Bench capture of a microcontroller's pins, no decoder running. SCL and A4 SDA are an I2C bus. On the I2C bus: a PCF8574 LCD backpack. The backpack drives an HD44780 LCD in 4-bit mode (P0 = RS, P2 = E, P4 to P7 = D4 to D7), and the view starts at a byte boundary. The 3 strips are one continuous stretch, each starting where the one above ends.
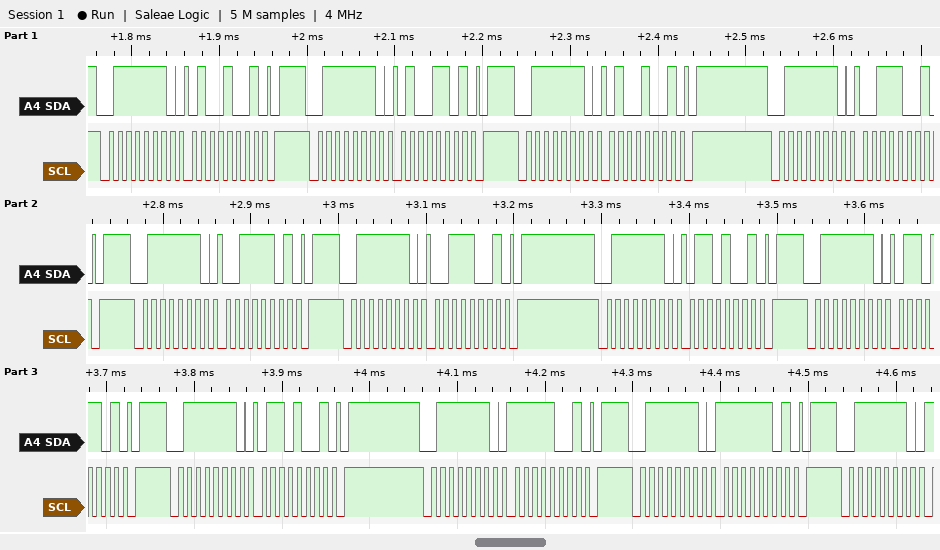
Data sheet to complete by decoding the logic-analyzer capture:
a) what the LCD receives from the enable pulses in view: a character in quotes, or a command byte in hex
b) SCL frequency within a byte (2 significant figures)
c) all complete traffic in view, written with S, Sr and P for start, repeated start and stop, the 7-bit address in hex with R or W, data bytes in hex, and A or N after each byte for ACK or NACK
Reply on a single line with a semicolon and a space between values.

'C'; 100 kHz; S 3FW A 49 A P S 3FW A 4D A P S 3FW A 49 A P S 3FW A 39 A P S 3FW A 3D A P S 3FW A 39 A P S 3FW A 69 A P S 3FW A 6D A P S 3FW A 69 A P S 3FW A F9 A P S 3FW A FD A P S 3FW A
